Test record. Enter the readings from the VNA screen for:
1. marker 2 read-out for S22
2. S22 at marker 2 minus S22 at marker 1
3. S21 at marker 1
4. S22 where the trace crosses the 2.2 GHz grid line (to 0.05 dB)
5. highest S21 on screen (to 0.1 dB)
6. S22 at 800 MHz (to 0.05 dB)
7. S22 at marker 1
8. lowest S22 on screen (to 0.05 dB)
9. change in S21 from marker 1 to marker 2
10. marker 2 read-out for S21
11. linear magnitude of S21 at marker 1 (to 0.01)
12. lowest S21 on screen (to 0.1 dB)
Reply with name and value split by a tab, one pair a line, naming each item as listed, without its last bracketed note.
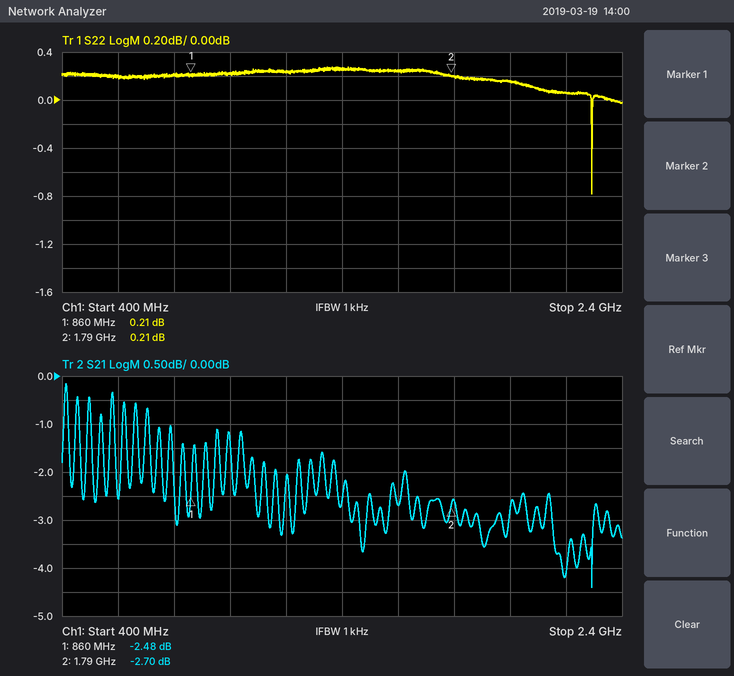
marker 2 read-out for S22	0.21 dB
S22 at marker 2 minus S22 at marker 1	0.00 dB
S21 at marker 1	-2.48 dB
S22 where the trace crosses the 2.2 GHz grid line	0.05 dB
highest S21 on screen	-0.2 dB
S22 at 800 MHz	0.20 dB
S22 at marker 1	0.21 dB
lowest S22 on screen	-0.80 dB
change in S21 from marker 1 to marker 2	-0.22 dB
marker 2 read-out for S21	-2.70 dB
linear magnitude of S21 at marker 1	0.75
lowest S21 on screen	-4.4 dB
